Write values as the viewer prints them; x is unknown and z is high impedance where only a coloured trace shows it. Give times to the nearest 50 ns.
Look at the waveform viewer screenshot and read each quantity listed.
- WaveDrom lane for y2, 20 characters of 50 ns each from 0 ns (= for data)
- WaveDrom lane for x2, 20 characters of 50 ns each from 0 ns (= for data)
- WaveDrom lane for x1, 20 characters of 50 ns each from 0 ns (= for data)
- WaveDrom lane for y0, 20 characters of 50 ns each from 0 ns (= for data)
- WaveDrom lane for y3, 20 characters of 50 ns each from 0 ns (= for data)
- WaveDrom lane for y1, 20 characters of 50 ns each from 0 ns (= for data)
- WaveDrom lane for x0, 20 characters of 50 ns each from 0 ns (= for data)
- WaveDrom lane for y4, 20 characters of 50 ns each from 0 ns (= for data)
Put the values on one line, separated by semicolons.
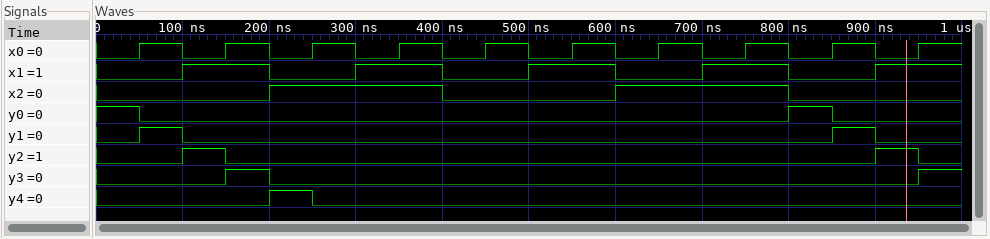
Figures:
{name: 'y2', wave: '0.10..............10'}; {name: 'x2', wave: '0...1...0...1...0...'}; {name: 'x1', wave: '0.1.0.1.0.1.0.1.0.1.'}; {name: 'y0', wave: '10..............10..'}; {name: 'y3', wave: '0..10..............1'}; {name: 'y1', wave: '010..............10.'}; {name: 'x0', wave: '01010101010101010101'}; {name: 'y4', wave: '0...10..............'}
